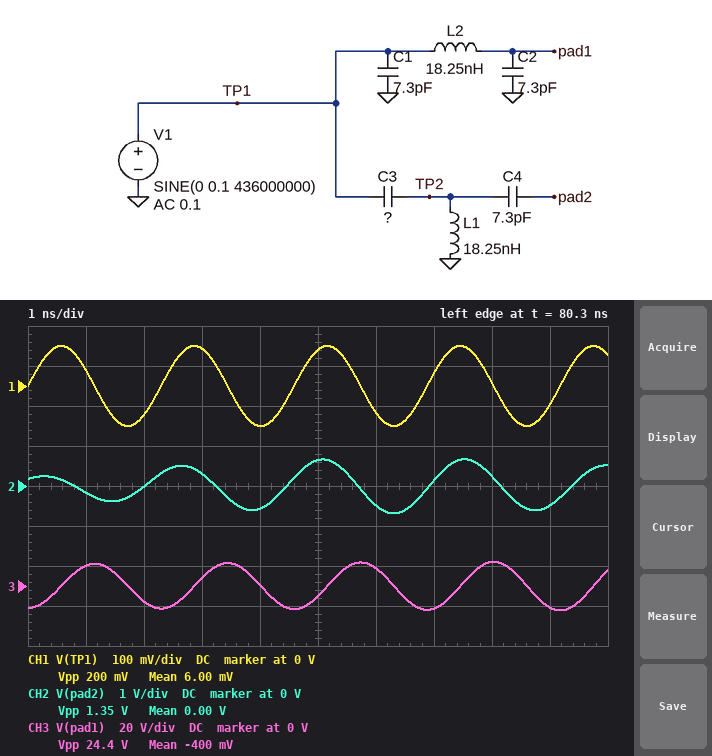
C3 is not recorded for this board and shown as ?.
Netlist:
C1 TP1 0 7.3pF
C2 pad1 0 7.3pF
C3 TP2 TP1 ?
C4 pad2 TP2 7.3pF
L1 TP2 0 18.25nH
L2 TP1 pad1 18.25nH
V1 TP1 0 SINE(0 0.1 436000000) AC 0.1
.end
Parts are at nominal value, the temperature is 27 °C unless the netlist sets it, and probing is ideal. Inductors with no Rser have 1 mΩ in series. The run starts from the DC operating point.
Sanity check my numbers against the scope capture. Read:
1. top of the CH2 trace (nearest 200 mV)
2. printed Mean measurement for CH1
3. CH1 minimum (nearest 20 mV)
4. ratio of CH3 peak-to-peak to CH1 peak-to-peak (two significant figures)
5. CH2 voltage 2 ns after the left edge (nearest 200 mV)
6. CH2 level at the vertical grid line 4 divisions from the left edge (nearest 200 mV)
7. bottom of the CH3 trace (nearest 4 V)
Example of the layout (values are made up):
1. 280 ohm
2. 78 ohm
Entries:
1. 600 mV
2. 6.00 mV
3. -100 mV
4. 120
5. 0 V
6. -600 mV
7. -12 V
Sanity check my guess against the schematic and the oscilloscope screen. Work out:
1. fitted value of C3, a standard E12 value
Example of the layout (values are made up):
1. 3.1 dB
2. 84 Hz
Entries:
1. 10 pF
